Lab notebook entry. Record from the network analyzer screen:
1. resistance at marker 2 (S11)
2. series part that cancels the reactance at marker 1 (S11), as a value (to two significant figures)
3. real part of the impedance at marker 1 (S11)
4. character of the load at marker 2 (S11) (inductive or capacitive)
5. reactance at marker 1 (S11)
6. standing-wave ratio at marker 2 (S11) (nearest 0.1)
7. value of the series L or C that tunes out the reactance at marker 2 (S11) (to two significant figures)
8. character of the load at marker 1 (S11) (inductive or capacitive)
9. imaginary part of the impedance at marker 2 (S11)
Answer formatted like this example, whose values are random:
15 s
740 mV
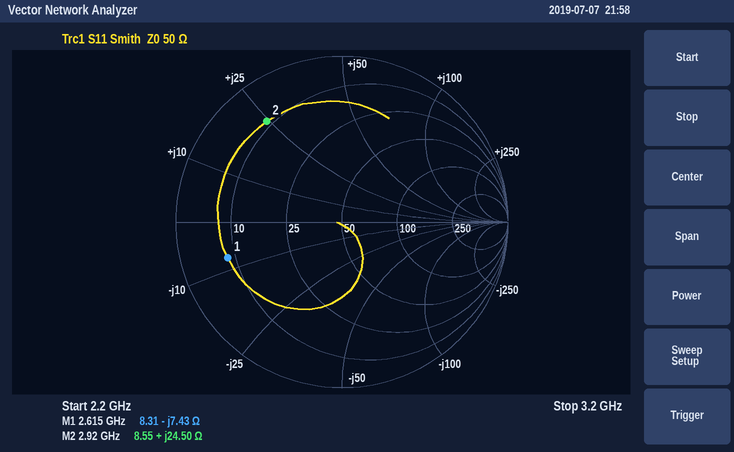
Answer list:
8.55 Ω
450 pH
8.31 Ω
inductive
-7.43 Ω
7.3
2.2 pF
capacitive
+24.50 Ω
